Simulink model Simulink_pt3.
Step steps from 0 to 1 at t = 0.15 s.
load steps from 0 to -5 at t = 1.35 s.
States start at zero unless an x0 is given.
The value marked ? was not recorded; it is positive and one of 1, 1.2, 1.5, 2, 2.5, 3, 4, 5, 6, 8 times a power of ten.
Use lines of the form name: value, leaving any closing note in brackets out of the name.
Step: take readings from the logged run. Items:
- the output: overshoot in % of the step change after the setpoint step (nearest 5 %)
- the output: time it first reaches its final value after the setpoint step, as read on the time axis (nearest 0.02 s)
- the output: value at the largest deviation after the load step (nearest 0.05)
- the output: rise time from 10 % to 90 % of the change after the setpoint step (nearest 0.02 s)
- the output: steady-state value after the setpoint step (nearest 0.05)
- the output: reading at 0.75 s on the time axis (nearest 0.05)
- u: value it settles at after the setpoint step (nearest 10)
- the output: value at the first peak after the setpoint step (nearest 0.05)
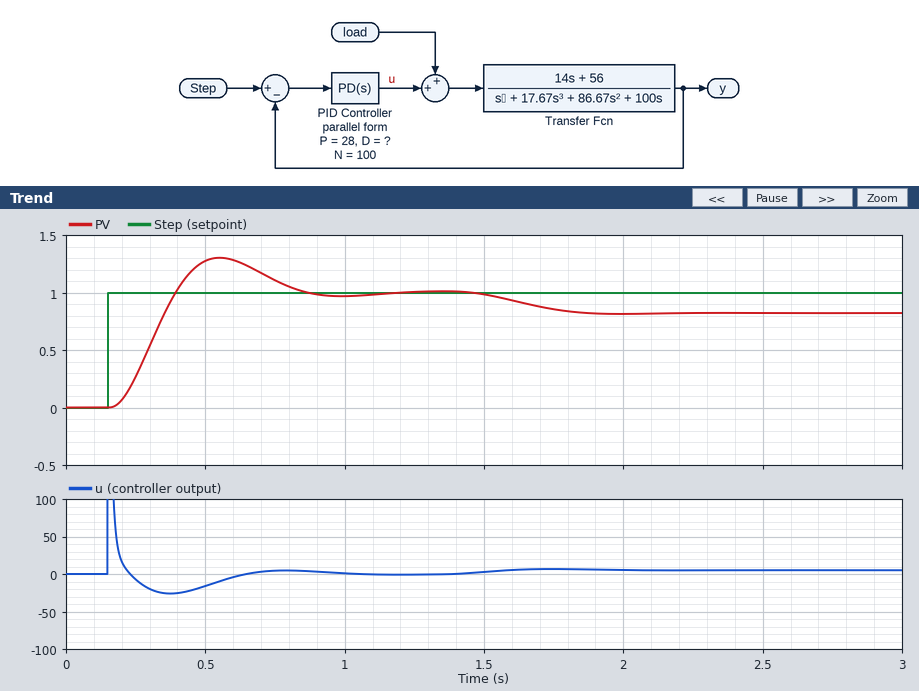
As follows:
the output: overshoot in % of the step change after the setpoint step: 30 %
the output: time it first reaches its final value after the setpoint step, as read on the time axis: 0.40 s
the output: value at the largest deviation after the load step: 0.80
the output: rise time from 10 % to 90 % of the change after the setpoint step: 0.16 s
the output: steady-state value after the setpoint step: 1.00
the output: reading at 0.75 s on the time axis: 1.10
u: value it settles at after the setpoint step: 0
the output: value at the first peak after the setpoint step: 1.30
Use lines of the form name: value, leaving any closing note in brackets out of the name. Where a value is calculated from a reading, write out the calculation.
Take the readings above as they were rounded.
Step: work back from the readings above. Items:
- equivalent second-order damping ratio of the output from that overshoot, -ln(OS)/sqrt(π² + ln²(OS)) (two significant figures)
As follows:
equivalent second-order damping ratio of the output from that overshoot, -ln(OS)/sqrt(π² + ln²(OS)): ln(0.3) = -1.204; 1.204 / sqrt(9.870 + 1.450) = 0.36
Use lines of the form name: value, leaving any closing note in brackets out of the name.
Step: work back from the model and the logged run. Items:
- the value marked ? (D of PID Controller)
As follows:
the value marked ?: 6
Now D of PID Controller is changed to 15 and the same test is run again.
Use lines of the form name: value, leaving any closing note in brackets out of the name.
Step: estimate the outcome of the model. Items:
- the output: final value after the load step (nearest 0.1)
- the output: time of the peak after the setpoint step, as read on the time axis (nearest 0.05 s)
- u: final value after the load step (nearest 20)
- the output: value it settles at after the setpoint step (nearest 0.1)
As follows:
the output: final value after the load step: 0.8
the output: time of the peak after the setpoint step, as read on the time axis: 0.40 s
u: final value after the load step: 0
the output: value it settles at after the setpoint step: 1.0
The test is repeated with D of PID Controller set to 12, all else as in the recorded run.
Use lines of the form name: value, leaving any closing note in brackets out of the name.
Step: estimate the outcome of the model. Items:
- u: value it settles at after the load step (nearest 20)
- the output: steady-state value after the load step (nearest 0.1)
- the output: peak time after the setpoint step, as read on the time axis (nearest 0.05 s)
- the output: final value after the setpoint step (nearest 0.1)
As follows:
u: value it settles at after the load step: 0
the output: steady-state value after the load step: 0.8
the output: peak time after the setpoint step, as read on the time axis: 0.40 s
the output: final value after the setpoint step: 1.0
